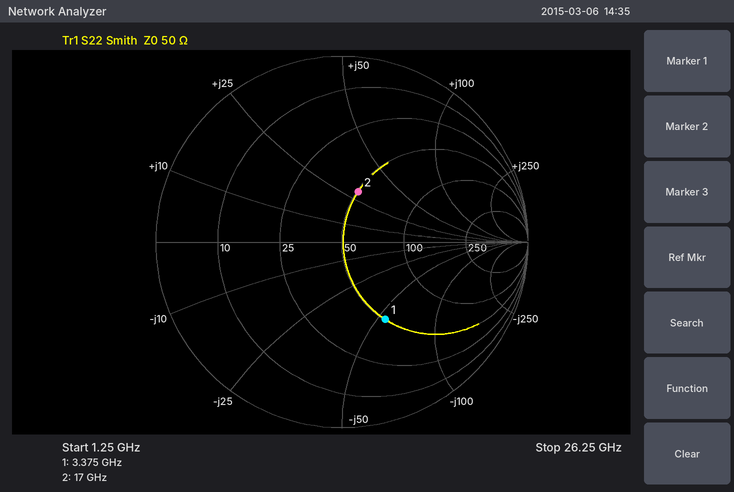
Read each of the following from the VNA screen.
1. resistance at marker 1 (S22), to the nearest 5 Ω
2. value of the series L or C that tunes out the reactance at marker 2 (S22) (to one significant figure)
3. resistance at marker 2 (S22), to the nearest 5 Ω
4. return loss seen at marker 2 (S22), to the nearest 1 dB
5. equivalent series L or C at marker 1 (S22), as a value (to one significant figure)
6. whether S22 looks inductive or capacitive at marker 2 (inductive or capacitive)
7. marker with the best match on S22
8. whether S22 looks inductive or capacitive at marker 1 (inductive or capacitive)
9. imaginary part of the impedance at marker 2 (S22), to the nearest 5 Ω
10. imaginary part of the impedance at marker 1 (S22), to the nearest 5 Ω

50 Ω
300 fF
50 Ω
11 dB
900 fF
inductive
marker 2
capacitive
+30 Ω
-55 Ω
